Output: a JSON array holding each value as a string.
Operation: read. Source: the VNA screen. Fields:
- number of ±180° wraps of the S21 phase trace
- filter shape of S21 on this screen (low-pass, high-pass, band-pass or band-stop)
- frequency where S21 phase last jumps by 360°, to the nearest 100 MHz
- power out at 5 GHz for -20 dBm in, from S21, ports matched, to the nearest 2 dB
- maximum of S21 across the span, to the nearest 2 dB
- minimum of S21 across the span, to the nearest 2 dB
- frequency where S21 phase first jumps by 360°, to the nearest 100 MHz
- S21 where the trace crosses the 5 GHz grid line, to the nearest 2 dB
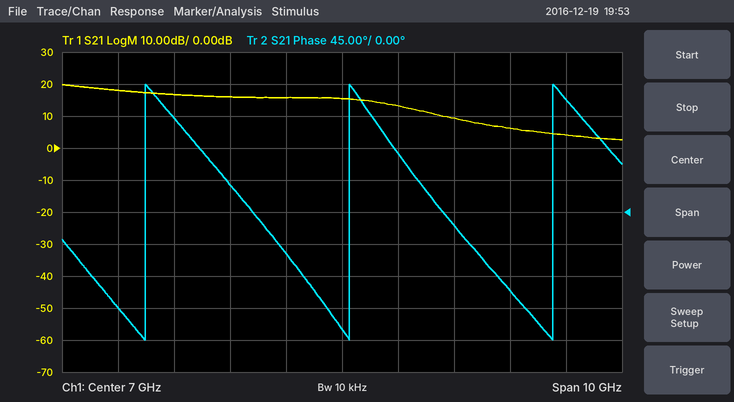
["3", "low-pass", "10.8 GHz", "-4 dBm", "20 dB", "2 dB", "3.5 GHz", "16 dB"]
